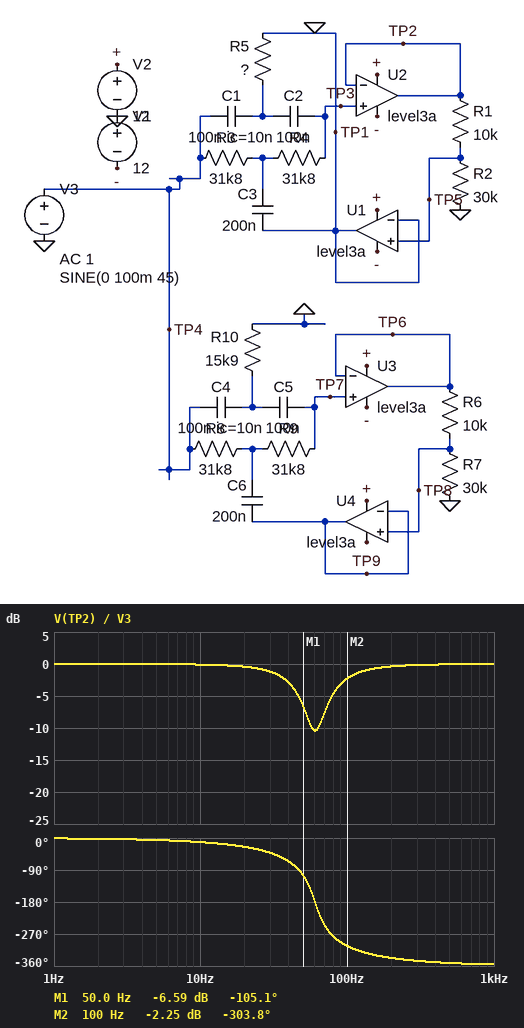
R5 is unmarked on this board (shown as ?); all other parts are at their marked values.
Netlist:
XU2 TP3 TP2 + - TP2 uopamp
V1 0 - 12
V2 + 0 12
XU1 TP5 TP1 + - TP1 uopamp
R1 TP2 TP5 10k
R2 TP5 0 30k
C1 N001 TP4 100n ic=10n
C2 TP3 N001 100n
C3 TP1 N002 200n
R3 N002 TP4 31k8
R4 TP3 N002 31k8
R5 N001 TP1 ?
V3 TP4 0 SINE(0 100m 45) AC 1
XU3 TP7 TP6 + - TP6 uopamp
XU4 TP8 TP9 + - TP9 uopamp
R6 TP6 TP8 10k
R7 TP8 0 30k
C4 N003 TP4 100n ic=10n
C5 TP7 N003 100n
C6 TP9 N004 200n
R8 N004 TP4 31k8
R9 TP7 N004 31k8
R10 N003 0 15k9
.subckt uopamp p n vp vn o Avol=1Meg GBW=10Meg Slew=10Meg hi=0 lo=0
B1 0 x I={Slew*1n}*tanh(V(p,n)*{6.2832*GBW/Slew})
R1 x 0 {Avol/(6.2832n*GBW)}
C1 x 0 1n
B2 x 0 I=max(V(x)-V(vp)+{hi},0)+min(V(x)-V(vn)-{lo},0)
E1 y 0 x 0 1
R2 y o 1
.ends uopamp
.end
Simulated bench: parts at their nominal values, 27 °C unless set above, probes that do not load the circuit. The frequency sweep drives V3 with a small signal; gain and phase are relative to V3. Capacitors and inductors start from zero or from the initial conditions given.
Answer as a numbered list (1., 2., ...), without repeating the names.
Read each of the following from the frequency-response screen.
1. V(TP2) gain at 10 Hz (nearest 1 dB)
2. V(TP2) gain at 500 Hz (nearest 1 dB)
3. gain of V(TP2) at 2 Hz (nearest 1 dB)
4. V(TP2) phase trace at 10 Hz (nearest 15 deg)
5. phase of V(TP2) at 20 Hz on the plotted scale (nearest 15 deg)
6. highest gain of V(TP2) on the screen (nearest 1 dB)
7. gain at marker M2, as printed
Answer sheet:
1. 0 dB
2. 0 dB
3. 0 dB
4. -15 deg
5. -30 deg
6. 0 dB
7. -2.25 dB
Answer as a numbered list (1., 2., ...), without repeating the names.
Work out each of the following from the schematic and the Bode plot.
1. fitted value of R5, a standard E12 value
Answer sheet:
1. 8.2 kΩ
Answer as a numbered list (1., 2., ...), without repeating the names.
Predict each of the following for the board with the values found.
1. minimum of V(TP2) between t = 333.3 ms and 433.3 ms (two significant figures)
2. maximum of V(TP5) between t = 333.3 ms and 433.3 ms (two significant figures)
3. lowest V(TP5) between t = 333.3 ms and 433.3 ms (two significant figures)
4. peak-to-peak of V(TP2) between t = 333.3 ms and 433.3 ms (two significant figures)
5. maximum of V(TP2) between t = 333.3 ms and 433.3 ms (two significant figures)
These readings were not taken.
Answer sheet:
1. -60 mV
2. 45 mV
3. -45 mV
4. 120 mV
5. 60 mV
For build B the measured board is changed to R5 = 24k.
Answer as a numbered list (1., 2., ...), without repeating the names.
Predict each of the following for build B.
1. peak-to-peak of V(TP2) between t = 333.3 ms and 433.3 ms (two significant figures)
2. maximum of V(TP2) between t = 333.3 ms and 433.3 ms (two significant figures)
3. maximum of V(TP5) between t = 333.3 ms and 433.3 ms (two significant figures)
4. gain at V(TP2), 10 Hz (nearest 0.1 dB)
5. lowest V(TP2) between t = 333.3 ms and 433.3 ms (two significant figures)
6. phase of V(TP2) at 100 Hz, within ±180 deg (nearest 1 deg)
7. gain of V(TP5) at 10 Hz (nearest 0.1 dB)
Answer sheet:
1. 40 mV
2. 20 mV
3. 15 mV
4. -0.3 dB
5. -20 mV
6. 26 deg
7. -2.8 dB
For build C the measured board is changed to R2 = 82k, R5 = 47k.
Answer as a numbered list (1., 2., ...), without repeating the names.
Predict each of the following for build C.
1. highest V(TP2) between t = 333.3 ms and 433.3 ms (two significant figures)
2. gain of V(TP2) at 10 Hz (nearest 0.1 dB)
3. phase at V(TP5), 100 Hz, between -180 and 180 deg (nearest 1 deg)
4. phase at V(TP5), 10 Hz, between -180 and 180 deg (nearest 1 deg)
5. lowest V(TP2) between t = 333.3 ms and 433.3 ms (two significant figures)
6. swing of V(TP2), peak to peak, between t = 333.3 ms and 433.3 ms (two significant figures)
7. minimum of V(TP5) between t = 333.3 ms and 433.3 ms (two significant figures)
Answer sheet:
1. 65 mV
2. -0.2 dB
3. 9 deg
4. -5 deg
5. -65 mV
6. 130 mV
7. -58 mV
